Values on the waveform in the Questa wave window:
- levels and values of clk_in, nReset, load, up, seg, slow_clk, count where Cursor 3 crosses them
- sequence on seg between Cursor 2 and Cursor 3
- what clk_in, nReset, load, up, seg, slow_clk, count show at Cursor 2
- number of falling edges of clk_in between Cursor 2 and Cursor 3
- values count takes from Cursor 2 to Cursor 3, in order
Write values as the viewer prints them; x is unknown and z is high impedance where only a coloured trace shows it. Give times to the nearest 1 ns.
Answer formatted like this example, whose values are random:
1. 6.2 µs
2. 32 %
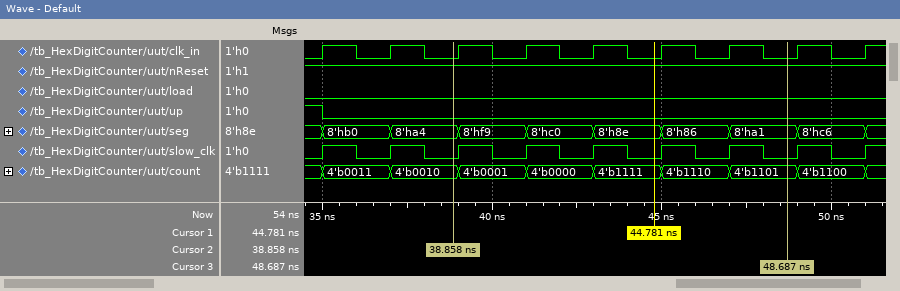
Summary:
1. clk_in=0, nReset=1, load=0, up=0, seg=8'ha1, slow_clk=0, count=4'b1101
2. 8'ha4, 8'hf9, 8'hc0, 8'h8e, 8'h86, 8'ha1
3. clk_in=0, nReset=1, load=0, up=0, seg=8'ha4, slow_clk=0, count=4'b0010
4. 5
5. 4'b0010, 4'b0001, 4'b0000, 4'b1111, 4'b1110, 4'b1101
